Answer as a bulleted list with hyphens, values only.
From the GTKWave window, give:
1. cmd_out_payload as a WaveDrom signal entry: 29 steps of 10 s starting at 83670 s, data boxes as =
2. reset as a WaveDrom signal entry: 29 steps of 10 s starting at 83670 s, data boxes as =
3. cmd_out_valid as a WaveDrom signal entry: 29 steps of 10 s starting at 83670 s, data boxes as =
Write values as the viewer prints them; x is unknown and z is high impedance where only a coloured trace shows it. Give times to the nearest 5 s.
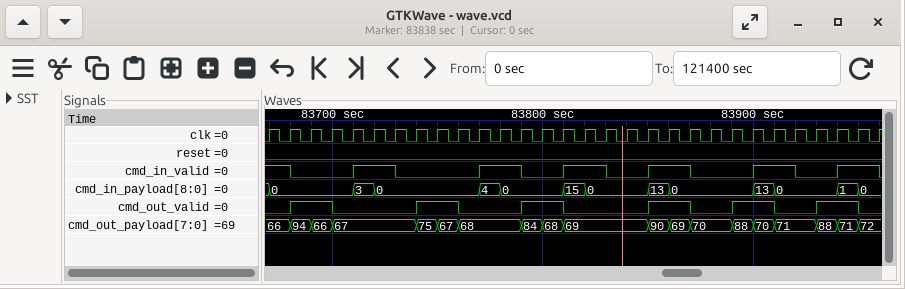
- {name: 'cmd_out_payload', wave: '====...===..===...===.===.===', data: '66 94 66 67 75 67 68 84 68 69 90 69 70 88 70 71 88 71 72'}
- {name: 'reset', wave: '0............................'}
- {name: 'cmd_out_valid', wave: '01.0...1.0..1.0...1.0.1.0.1.0'}
